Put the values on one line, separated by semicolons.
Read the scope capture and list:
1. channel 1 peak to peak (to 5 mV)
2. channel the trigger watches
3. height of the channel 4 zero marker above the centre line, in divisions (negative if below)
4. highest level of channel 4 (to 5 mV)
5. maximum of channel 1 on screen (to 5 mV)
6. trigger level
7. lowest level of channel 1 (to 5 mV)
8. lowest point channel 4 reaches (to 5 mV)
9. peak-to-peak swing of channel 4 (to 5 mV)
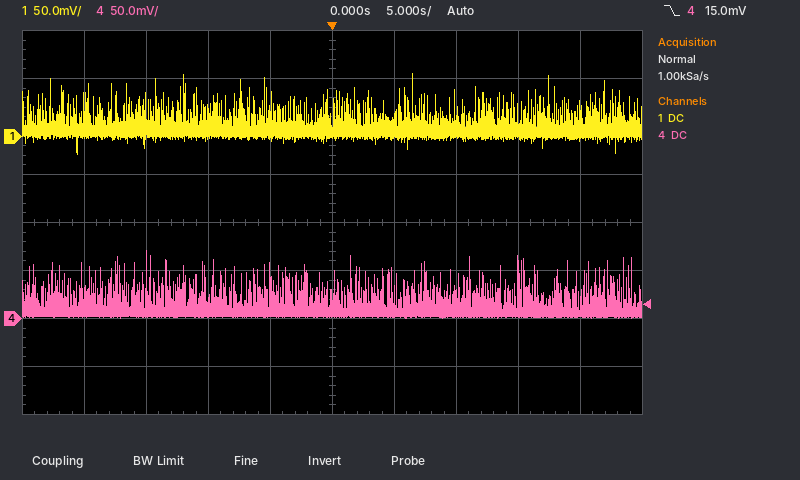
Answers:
85 mV; channel 4; -2.0 div; 70 mV; 65 mV; 15.0 mV; -20 mV; 0 mV; 70 mV
